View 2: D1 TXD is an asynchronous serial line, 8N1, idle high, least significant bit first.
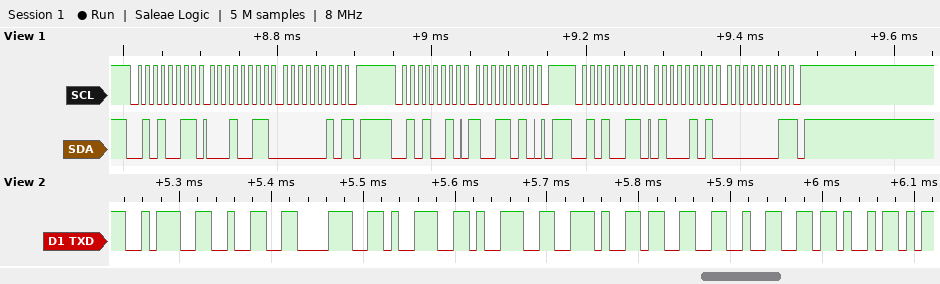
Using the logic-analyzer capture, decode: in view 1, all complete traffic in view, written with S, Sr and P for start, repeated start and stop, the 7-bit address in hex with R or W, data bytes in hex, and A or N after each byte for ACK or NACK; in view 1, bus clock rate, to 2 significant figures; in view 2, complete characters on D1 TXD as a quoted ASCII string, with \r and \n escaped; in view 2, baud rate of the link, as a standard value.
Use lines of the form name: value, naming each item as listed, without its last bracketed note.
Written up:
in view 1, all complete traffic in view, written with S, Sr and P for start, repeated start and stop, the 7-bit address in hex with R or W, data bytes in hex, and A or N after each byte for ACK or NACK: S 29R A 13 A 02 N P S 29W A 9A A P S 29R A 45 A 01 N P
in view 1, bus clock rate, to 2 significant figures: 100 kHz
in view 2, complete characters on D1 TXD as a quoted ASCII string, with \r and \n escaped: ":2899.32K"
in view 2, baud rate of the link, as a standard value: 115200 baud
